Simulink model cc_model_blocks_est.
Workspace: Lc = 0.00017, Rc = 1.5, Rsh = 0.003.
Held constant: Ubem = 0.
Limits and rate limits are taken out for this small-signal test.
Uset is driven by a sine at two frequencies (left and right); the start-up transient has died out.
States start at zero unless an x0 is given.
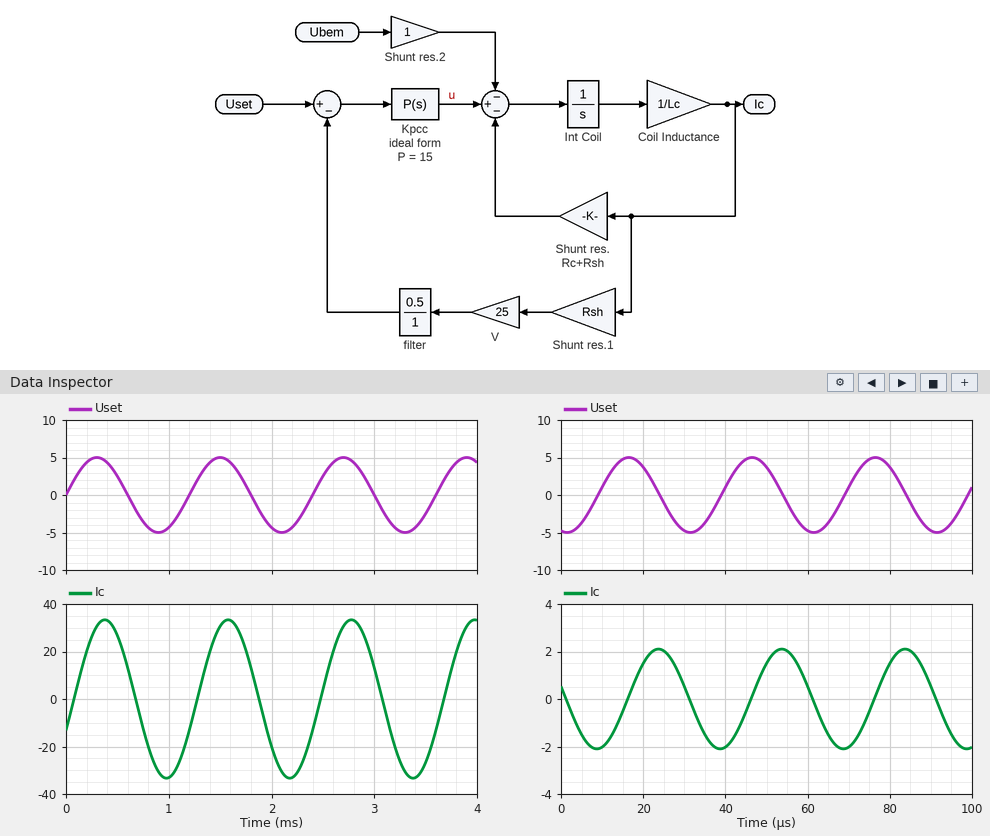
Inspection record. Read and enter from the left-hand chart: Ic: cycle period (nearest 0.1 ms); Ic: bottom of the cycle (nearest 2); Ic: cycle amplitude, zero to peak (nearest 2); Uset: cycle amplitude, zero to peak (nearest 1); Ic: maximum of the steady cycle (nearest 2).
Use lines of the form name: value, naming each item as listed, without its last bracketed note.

Ic: cycle period: 1.2 ms
Ic: bottom of the cycle: -34
Ic: cycle amplitude, zero to peak: 34
Uset: cycle amplitude, zero to peak: 5
Ic: maximum of the steady cycle: 34
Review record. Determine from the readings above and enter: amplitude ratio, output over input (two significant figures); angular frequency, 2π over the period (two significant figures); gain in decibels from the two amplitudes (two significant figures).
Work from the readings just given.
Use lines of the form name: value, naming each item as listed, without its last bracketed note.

amplitude ratio, output over input: 6.8
angular frequency, 2π over the period: 5.2 rad/ms
gain in decibels from the two amplitudes: 17 dB
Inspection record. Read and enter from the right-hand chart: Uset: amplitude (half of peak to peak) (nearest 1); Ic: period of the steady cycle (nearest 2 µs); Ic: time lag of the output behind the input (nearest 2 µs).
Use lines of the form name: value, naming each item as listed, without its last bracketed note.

Uset: amplitude (half of peak to peak): 5
Ic: period of the steady cycle: 30 µs
Ic: time lag of the output behind the input: 8 µs
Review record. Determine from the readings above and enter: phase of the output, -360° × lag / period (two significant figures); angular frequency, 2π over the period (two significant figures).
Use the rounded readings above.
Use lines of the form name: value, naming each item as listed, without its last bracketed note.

phase of the output, -360° × lag / period: -96°
angular frequency, 2π over the period: 0.21 rad/µs
